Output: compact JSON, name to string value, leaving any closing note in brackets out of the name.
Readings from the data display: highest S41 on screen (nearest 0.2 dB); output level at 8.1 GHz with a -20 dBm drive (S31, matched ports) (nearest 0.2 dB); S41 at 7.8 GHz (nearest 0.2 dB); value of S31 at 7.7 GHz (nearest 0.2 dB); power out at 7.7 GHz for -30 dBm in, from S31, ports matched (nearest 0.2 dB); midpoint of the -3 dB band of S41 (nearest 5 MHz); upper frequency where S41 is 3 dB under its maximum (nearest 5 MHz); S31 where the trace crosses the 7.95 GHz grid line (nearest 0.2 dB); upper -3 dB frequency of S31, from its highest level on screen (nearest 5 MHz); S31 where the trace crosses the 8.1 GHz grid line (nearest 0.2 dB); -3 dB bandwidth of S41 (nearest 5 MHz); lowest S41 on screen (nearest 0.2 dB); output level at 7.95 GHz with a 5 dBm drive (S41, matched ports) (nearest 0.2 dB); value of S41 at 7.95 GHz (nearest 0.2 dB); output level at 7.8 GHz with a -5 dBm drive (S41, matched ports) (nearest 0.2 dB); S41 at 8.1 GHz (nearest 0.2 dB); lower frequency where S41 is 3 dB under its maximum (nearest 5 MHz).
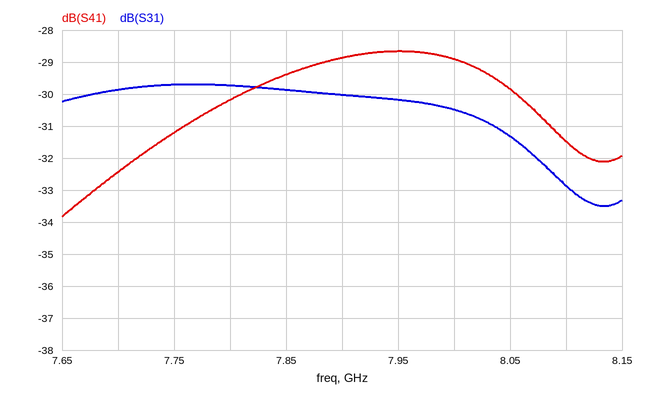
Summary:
{"highest S41 on screen": "-28.6 dB", "output level at 8.1 GHz with a -20 dBm drive (S31, matched ports)": "-52.8 dBm", "S41 at 7.8 GHz": "-30.2 dB", "value of S31 at 7.7 GHz": "-29.8 dB", "power out at 7.7 GHz for -30 dBm in, from S31, ports matched": "-59.8 dBm", "midpoint of the -3 dB band of S41": "7.920 GHz", "upper frequency where S41 is 3 dB under its maximum": "8.105 GHz", "S31 where the trace crosses the 7.95 GHz grid line": "-30.2 dB", "upper -3 dB frequency of S31, from its highest level on screen": "8.095 GHz", "S31 where the trace crosses the 8.1 GHz grid line": "-32.8 dB", "-3 dB bandwidth of S41": "375 MHz", "lowest S41 on screen": "-33.8 dB", "output level at 7.95 GHz with a 5 dBm drive (S41, matched ports)": "-23.6 dBm", "value of S41 at 7.95 GHz": "-28.6 dB", "output level at 7.8 GHz with a -5 dBm drive (S41, matched ports)": "-35.2 dBm", "S41 at 8.1 GHz": "-31.4 dB", "lower frequency where S41 is 3 dB under its maximum": "7.730 GHz"}
